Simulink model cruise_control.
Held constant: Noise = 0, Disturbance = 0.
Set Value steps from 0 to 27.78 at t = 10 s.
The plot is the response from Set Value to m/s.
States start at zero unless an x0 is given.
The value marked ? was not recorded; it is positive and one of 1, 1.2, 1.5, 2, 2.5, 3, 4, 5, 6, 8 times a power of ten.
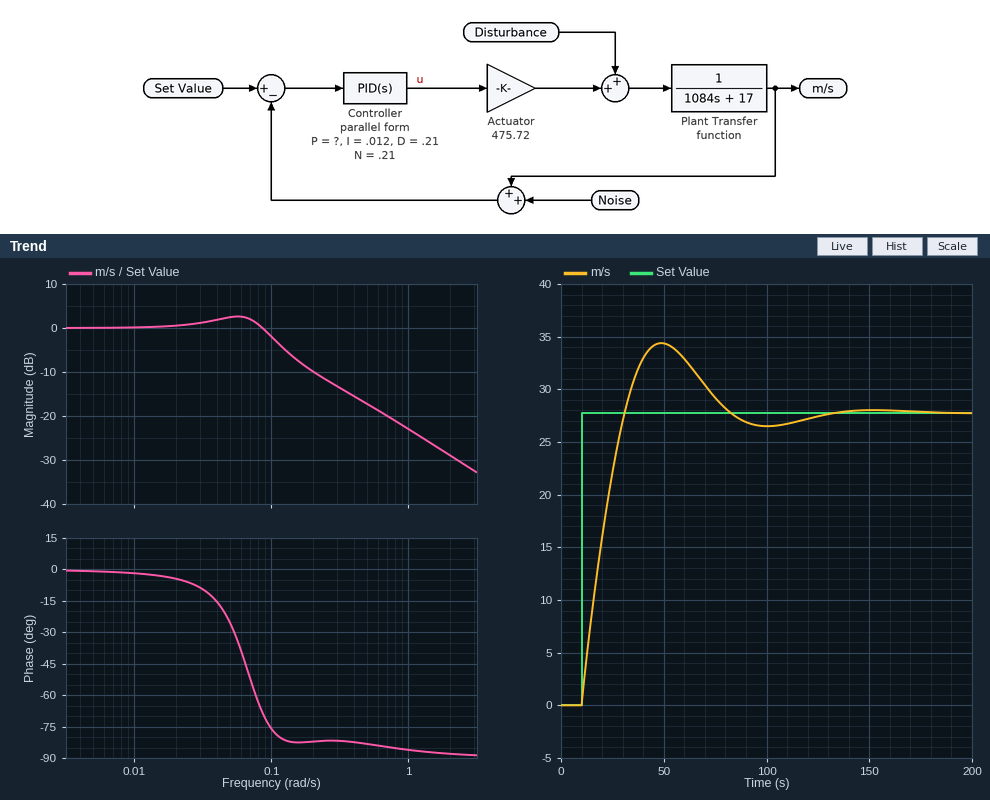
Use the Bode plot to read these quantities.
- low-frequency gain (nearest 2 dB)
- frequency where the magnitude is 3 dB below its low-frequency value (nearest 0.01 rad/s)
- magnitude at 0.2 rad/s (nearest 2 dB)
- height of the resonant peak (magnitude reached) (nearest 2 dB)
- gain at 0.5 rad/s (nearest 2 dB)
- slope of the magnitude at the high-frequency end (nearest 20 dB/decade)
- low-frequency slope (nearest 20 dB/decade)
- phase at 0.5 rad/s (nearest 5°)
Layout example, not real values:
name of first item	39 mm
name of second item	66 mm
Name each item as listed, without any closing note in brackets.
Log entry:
low-frequency gain	0 dB
frequency where the magnitude is 3 dB below its low-frequency value	0.11 rad/s
magnitude at 0.2 rad/s	-10 dB
height of the resonant peak (magnitude reached)	2 dB
gain at 0.5 rad/s	-18 dB
slope of the magnitude at the high-frequency end	-20 dB/decade
low-frequency slope	0 dB/decade
phase at 0.5 rad/s	-85°
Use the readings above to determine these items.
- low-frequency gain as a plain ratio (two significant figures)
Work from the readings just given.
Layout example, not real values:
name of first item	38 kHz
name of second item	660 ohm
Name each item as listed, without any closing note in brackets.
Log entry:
low-frequency gain as a plain ratio	1.0
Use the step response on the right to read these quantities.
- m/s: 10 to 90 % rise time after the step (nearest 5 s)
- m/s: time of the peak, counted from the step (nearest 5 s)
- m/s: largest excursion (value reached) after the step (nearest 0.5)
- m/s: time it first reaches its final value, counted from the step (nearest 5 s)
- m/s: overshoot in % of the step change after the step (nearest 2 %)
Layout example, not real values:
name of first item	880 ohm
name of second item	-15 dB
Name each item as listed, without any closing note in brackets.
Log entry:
m/s: 10 to 90 % rise time after the step	15 s
m/s: time of the peak, counted from the step	40 s
m/s: largest excursion (value reached) after the step	34.5
m/s: time it first reaches its final value, counted from the step	20 s
m/s: overshoot in % of the step change after the step	24 %
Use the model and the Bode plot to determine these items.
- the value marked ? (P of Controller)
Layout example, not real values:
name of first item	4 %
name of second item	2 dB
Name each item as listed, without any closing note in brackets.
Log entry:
the value marked ?	0.12
